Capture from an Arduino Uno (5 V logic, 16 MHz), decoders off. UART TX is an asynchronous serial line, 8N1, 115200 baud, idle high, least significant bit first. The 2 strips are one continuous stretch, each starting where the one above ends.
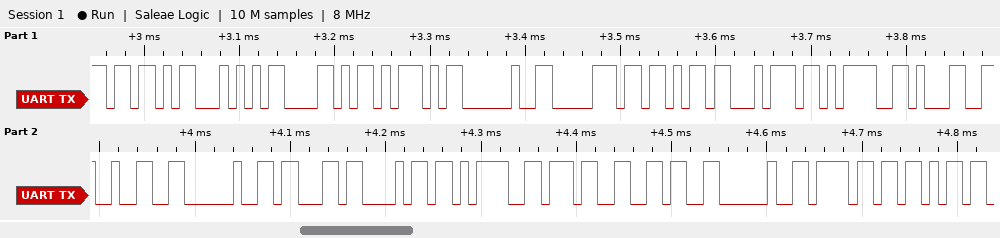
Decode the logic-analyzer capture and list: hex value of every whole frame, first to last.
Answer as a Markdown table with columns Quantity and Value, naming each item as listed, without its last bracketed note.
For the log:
| Quantity | Value |
|---|---|
| hex value of every whole frame, first to last | 0x5B 0x54 0x58 0x5D 0x20 0x70 0x6B 0x74 0x3D 0x31 0x32 0x20 0x63 0x68 0x3D 0x37 0x36 0x20 0x6F 0x6B |
